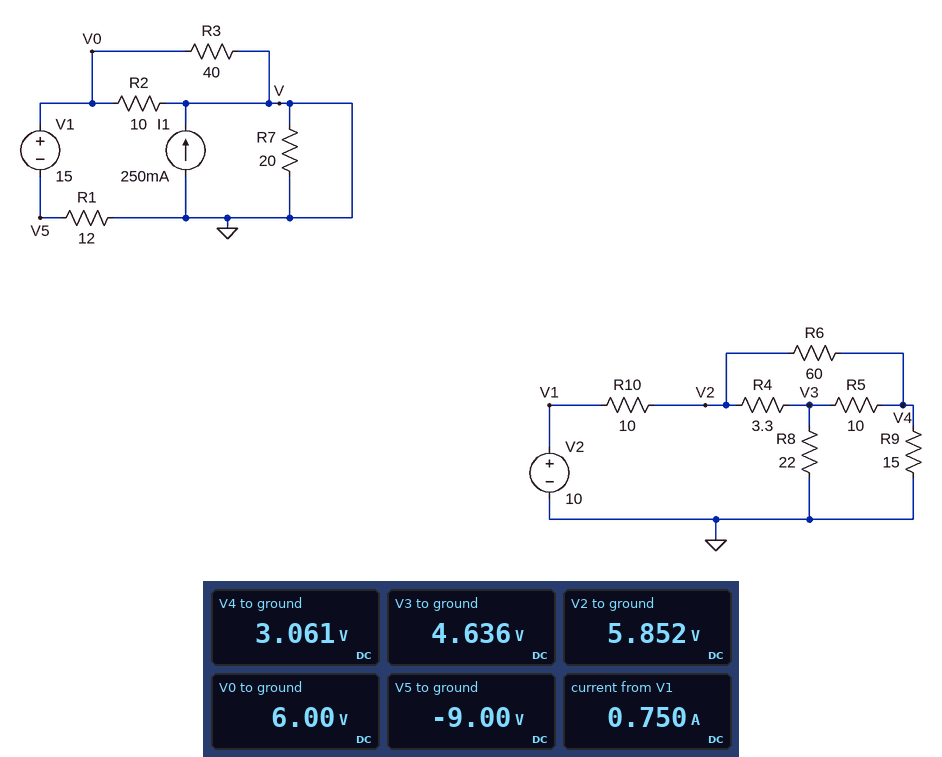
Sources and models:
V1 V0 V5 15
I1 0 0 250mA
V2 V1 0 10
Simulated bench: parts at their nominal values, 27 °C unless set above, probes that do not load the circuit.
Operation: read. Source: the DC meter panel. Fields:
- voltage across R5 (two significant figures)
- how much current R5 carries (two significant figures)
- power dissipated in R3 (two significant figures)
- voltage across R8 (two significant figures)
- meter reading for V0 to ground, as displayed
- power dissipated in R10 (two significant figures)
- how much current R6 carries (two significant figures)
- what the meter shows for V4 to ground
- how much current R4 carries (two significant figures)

1.6 V
160 mA
900 mW
4.6 V
6.00 V
1.7 W
47 mA
3.061 V
370 mA
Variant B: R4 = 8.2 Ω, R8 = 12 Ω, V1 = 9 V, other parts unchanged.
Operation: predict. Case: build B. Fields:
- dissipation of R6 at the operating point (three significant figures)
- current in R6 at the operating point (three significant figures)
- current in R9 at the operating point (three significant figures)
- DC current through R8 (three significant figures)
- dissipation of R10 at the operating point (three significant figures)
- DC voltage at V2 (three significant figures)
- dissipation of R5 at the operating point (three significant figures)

228 mW
61.7 mA
149 mA
258 mA
1.66 W
5.93 V
75.6 mW
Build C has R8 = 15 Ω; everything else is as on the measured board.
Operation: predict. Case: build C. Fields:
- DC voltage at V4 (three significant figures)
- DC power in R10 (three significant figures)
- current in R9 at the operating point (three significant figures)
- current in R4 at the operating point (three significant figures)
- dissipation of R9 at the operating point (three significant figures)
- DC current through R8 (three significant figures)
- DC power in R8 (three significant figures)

2.73 V
2.07 W
182 mA
410 mA
497 mW
273 mA
1.12 W
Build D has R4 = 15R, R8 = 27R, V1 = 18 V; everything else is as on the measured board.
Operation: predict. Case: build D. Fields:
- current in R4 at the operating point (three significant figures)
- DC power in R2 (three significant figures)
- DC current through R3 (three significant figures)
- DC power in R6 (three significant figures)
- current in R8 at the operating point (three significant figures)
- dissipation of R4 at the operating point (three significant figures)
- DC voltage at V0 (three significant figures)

229 mA
5.18 W
180 mA
324 mW
131 mA
786 mW
7.20 V
